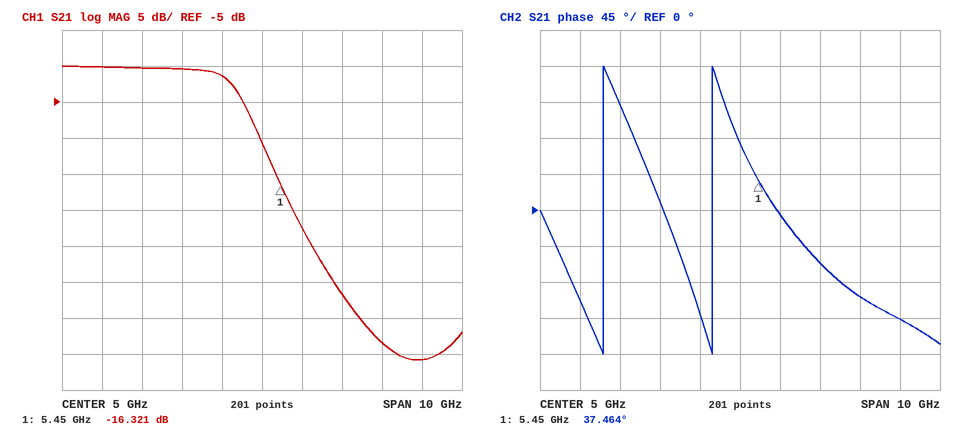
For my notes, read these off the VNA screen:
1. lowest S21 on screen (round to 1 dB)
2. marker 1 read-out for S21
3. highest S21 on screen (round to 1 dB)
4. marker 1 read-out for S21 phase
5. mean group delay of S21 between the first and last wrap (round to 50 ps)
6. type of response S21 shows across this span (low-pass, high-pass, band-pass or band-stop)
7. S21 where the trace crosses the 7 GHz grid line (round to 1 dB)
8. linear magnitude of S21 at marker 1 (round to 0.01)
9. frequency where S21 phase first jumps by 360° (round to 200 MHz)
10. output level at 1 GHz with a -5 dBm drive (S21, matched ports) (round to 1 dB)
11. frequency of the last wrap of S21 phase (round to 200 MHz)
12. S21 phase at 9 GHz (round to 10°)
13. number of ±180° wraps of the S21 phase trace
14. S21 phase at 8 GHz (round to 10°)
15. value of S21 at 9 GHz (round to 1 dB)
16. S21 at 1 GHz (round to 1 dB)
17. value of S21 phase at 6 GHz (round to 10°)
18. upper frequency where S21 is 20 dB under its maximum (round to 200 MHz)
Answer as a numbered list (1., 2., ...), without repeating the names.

1. -41 dB
2. -16.321 dB
3. 0 dB
4. 37.464°
5. 350 ps
6. low-pass
7. -32 dB
8. 0.15
9. 1.6 GHz
10. -5 dBm
11. 4.4 GHz
12. -140°
13. 2
14. -110°
15. -41 dB
16. 0 dB
17. -10°
18. 5.8 GHz
